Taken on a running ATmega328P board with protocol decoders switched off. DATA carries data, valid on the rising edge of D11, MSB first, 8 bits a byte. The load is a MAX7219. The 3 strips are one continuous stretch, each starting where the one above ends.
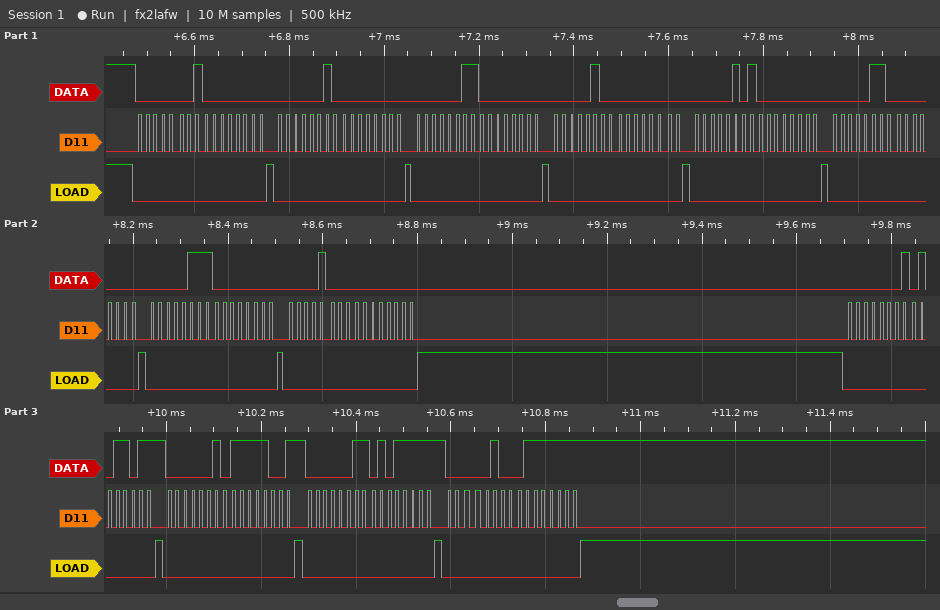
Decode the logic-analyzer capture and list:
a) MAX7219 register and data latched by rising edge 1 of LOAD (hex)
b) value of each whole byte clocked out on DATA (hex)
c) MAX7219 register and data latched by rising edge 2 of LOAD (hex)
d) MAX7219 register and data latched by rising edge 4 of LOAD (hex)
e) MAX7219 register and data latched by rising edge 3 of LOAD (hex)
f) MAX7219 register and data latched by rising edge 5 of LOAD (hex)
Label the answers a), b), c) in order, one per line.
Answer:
a) register 0x1, data 0x00
b) 01 00 02 00 03 00 04 00 05 00 06 00 07 00 08 00 01 5B 02 F9 03 5F 04 7F
c) register 0x2, data 0x00
d) register 0x4, data 0x00
e) register 0x3, data 0x00
f) register 0x5, data 0x00
